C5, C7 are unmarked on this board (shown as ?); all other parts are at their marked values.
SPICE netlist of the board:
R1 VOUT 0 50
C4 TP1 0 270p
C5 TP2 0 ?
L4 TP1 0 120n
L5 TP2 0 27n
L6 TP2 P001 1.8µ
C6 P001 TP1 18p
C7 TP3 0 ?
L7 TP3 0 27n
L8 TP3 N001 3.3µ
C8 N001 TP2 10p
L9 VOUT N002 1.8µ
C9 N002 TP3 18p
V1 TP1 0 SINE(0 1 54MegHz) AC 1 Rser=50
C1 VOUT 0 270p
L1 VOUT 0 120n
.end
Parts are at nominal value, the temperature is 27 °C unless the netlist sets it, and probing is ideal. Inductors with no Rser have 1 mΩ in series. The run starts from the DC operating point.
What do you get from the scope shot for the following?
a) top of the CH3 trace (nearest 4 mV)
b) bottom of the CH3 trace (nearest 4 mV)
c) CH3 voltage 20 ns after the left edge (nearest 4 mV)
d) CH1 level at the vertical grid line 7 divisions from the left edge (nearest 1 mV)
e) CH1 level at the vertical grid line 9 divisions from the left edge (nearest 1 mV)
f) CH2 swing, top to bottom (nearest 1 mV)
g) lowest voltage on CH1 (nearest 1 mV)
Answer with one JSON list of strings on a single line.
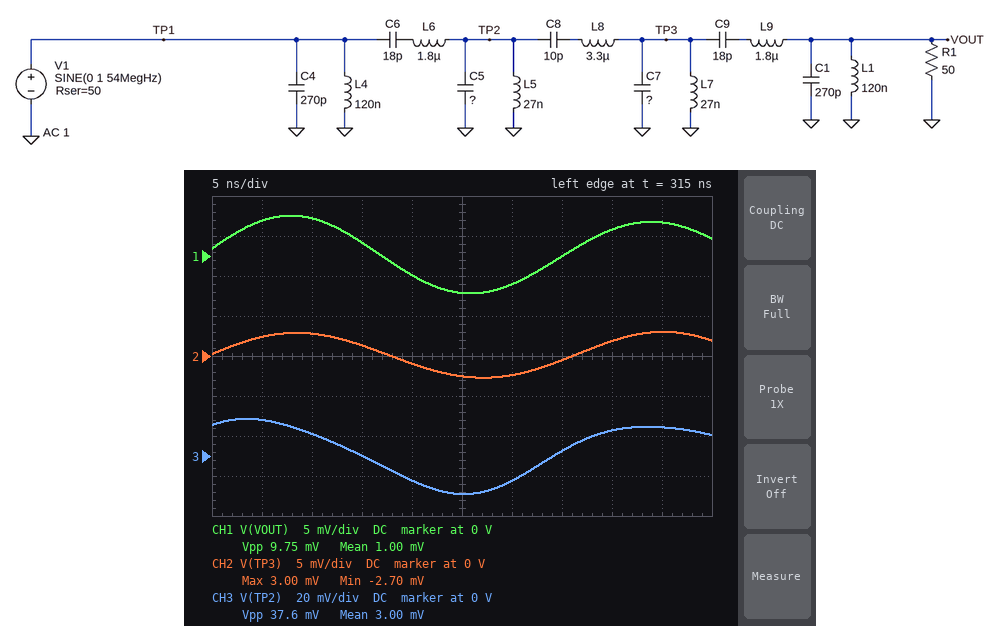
["20 mV", "-20 mV", "-12 mV", "0 V", "4 mV", "6 mV", "-5 mV"]
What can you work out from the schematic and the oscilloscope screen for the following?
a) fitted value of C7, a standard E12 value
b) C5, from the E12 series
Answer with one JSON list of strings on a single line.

["820 pF", "1.5 nF"]
